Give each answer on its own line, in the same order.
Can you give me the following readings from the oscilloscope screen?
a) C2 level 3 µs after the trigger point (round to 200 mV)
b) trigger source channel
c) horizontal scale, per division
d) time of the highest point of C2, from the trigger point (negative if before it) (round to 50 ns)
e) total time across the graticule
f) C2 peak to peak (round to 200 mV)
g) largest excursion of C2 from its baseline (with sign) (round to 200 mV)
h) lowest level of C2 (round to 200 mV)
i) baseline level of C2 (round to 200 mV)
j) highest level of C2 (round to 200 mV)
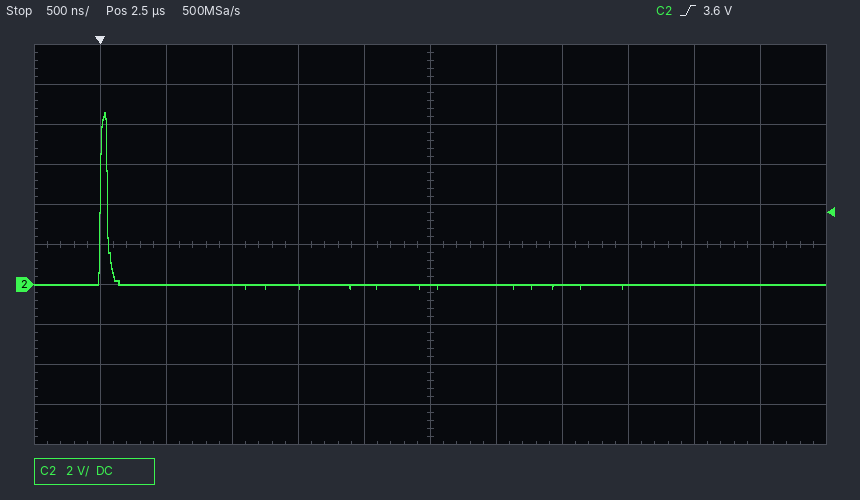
0.0 V
C2
500 ns
+50 ns
6 µs
8.8 V
+8.6 V
-200 mV
0.0 V
8.6 V
